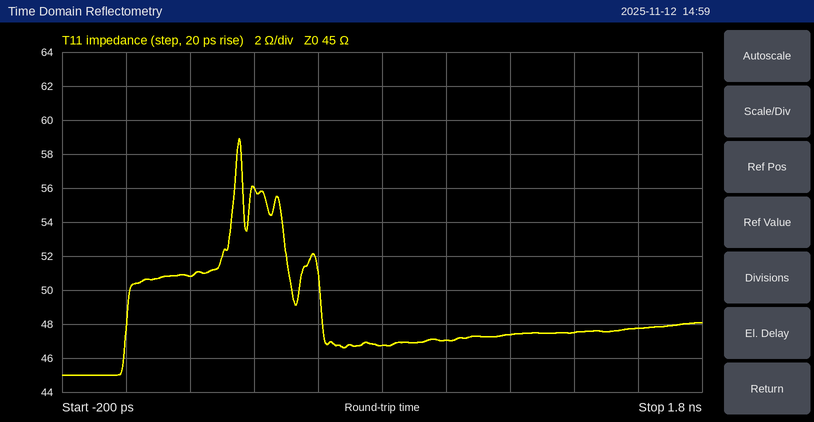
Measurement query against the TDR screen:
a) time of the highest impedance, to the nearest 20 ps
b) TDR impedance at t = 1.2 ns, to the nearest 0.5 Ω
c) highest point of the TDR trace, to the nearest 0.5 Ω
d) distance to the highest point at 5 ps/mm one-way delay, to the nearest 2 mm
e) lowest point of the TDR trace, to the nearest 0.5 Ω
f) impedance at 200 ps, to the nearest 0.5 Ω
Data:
360 ps
47.5 Ω
59.0 Ω
36 mm
45.0 Ω
51.0 Ω
